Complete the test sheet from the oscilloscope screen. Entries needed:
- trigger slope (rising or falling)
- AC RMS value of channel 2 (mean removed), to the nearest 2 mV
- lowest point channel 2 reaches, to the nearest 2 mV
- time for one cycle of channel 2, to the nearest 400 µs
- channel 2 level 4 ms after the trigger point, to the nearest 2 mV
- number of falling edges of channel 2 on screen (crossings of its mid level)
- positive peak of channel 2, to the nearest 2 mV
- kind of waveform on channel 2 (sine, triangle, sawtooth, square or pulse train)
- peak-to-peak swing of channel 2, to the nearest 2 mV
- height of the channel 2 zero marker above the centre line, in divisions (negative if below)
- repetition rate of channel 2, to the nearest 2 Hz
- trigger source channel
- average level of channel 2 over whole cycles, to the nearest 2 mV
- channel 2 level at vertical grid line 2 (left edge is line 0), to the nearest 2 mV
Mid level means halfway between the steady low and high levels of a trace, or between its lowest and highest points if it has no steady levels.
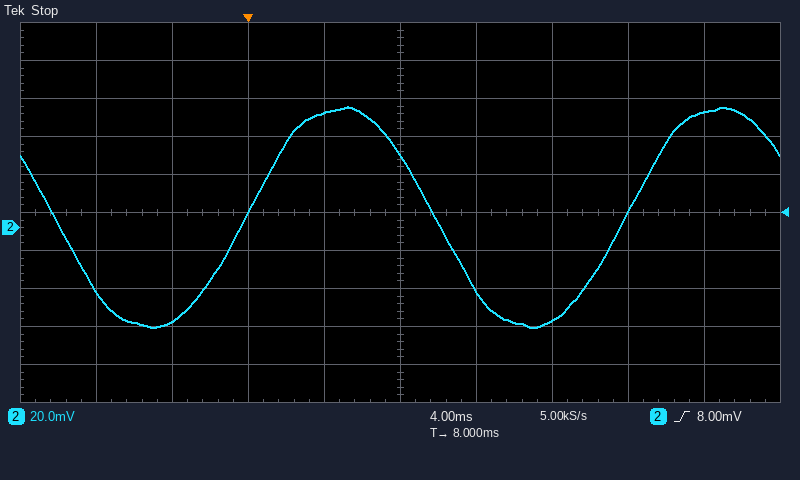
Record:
rising
42 mV
-52 mV
20.0 ms
60 mV
2
64 mV
sine
116 mV
-0.4 div
50 Hz
channel 2
6 mV
-50 mV
